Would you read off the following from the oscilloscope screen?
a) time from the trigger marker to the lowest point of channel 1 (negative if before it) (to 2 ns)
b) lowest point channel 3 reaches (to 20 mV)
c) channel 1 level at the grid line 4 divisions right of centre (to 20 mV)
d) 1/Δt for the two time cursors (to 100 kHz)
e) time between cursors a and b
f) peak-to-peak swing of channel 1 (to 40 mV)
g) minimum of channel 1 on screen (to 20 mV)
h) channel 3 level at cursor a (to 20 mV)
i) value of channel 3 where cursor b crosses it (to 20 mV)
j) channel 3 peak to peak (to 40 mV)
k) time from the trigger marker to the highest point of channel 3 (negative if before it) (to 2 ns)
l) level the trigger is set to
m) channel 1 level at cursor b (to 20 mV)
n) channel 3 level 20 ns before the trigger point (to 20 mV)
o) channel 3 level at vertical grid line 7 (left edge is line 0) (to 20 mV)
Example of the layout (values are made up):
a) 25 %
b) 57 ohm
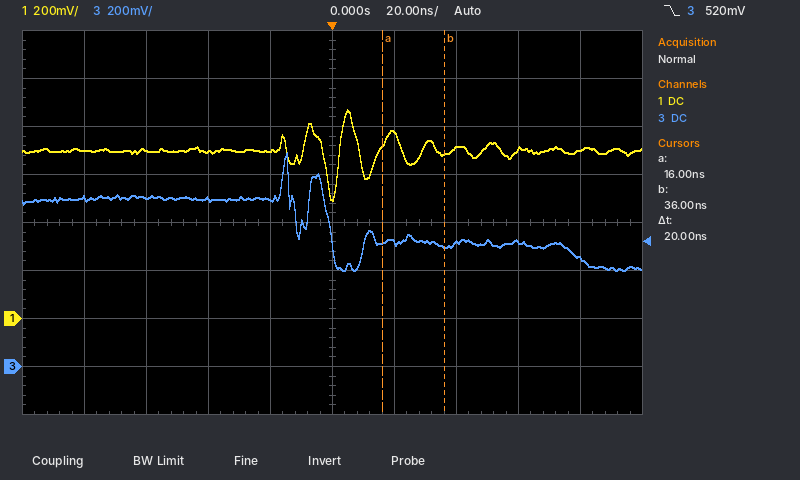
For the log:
a) 0 ns
b) 400 mV
c) 700 mV
d) 50.0 MHz
e) 20 ns
f) 360 mV
g) 500 mV
h) 520 mV
i) 500 mV
j) 480 mV
k) -14 ns
l) 520 mV
m) 680 mV
n) 700 mV
o) 520 mV
